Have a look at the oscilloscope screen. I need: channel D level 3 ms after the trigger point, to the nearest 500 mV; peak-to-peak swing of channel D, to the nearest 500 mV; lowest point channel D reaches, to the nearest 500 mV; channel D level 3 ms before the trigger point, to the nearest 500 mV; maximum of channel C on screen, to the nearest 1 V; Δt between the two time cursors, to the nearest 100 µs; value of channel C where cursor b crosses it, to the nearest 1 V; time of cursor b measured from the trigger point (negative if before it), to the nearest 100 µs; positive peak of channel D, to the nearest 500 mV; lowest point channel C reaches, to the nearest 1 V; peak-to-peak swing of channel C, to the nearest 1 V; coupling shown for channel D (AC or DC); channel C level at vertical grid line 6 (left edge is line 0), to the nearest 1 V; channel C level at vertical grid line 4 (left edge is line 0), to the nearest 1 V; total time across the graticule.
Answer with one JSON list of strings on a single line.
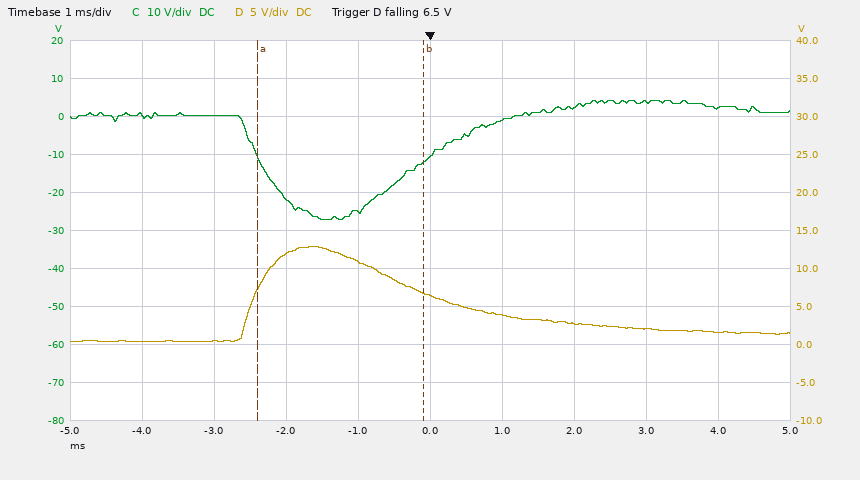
["2.0 V", "12.5 V", "500 mV", "500 mV", "4 V", "2.3 ms", "-12 V", "-100 µs", "13.0 V", "-27 V", "31 V", "DC", "-1 V", "-25 V", "10 ms"]
